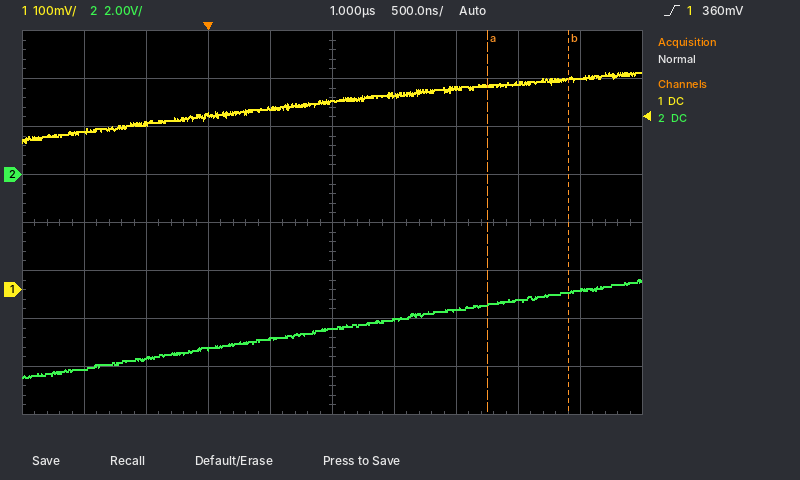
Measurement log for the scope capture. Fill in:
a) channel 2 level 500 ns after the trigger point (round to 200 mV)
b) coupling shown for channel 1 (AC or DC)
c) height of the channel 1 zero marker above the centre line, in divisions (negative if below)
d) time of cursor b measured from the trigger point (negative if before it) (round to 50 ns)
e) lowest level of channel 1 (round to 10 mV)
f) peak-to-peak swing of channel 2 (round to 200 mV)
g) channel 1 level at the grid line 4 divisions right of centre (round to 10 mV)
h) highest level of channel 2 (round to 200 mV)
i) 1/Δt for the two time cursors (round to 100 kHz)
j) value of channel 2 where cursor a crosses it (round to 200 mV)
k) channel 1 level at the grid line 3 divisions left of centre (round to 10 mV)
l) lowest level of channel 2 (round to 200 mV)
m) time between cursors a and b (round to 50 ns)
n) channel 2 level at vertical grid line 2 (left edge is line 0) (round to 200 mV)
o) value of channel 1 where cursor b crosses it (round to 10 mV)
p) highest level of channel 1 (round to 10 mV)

-6.8 V
DC
-1.4 div
+2.90 µs
310 mV
4.0 V
440 mV
-4.4 V
1.5 MHz
-5.4 V
350 mV
-8.4 V
650 ns
-7.6 V
440 mV
450 mV
